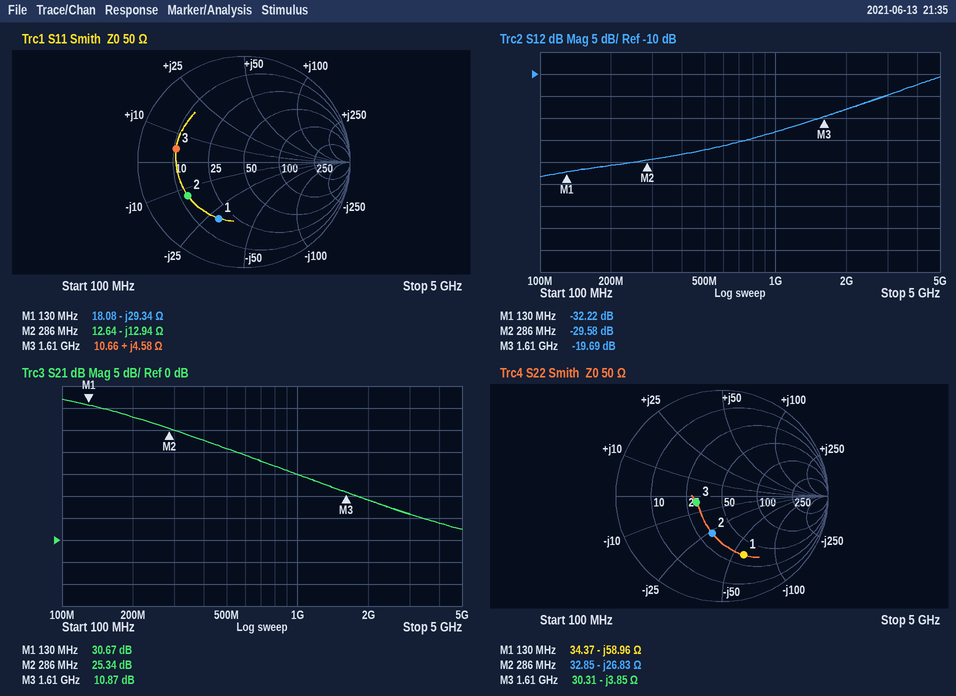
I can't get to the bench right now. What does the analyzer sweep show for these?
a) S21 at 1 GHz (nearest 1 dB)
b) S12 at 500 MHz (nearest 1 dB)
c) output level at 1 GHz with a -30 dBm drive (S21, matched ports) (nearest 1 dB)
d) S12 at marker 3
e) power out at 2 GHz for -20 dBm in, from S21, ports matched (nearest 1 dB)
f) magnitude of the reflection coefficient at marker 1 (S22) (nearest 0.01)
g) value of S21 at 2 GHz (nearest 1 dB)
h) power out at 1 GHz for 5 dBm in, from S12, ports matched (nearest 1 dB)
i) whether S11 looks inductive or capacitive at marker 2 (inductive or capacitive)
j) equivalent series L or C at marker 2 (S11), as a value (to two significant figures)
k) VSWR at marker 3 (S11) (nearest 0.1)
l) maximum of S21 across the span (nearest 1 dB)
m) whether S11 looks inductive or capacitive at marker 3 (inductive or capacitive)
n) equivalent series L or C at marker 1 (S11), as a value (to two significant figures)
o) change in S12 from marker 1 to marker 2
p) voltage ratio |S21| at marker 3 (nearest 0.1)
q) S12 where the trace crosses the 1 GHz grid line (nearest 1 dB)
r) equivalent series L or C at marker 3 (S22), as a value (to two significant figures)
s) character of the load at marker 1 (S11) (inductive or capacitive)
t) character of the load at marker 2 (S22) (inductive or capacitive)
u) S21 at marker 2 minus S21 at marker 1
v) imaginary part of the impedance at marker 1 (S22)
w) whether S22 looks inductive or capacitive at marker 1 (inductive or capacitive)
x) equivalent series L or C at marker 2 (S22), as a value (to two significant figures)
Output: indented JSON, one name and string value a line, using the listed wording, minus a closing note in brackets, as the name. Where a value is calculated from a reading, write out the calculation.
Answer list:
{
  "S21 at 1 GHz": "15 dB",
  "S12 at 500 MHz": "-27 dB",
  "output level at 1 GHz with a -30 dBm drive (S21, matched ports)": "-30 dBm + (15 dB) = -15 dBm",
  "S12 at marker 3": "-19.69 dB",
  "power out at 2 GHz for -20 dBm in, from S21, ports matched": "-20 dBm + (9 dB) = -11 dBm",
  "magnitude of the reflection coefficient at marker 1 (S22)": "0.59",
  "value of S21 at 2 GHz": "9 dB",
  "power out at 1 GHz for 5 dBm in, from S12, ports matched": "5 dBm + (-23 dB) = -18 dBm",
  "whether S11 looks inductive or capacitive at marker 2": "capacitive",
  "equivalent series L or C at marker 2 (S11), as a value": "C = 1/(2π × 286 MHz × 12.94 Ω) ≈ 43 pF",
  "VSWR at marker 3 (S11)": "4.7",
  "maximum of S21 across the span": "32 dB",
  "whether S11 looks inductive or capacitive at marker 3": "inductive",
  "equivalent series L or C at marker 1 (S11), as a value": "C = 1/(2π × 130 MHz × 29.34 Ω) ≈ 42 pF",
  "change in S12 from marker 1 to marker 2": "-29.58 − (-32.22) = 2.64 dB",
  "voltage ratio |S21| at marker 3": "10^(10.87/20) ≈ 3.5",
  "S12 where the trace crosses the 1 GHz grid line": "-23 dB",
  "equivalent series L or C at marker 3 (S22), as a value": "C = 1/(2π × 1.61 GHz × 3.85 Ω) ≈ 26 pF",
  "character of the load at marker 1 (S11)": "capacitive",
  "character of the load at marker 2 (S22)": "capacitive",
  "S21 at marker 2 minus S21 at marker 1": "25.34 − (30.67) = -5.33 dB",
  "imaginary part of the impedance at marker 1": "-58.96 Ω",
  "whether S22 looks inductive or capacitive at marker 1": "capacitive",
  "equivalent series L or C at marker 2 (S22), as a value": "C = 1/(2π × 286 MHz × 26.83 Ω) ≈ 21 pF"
}
